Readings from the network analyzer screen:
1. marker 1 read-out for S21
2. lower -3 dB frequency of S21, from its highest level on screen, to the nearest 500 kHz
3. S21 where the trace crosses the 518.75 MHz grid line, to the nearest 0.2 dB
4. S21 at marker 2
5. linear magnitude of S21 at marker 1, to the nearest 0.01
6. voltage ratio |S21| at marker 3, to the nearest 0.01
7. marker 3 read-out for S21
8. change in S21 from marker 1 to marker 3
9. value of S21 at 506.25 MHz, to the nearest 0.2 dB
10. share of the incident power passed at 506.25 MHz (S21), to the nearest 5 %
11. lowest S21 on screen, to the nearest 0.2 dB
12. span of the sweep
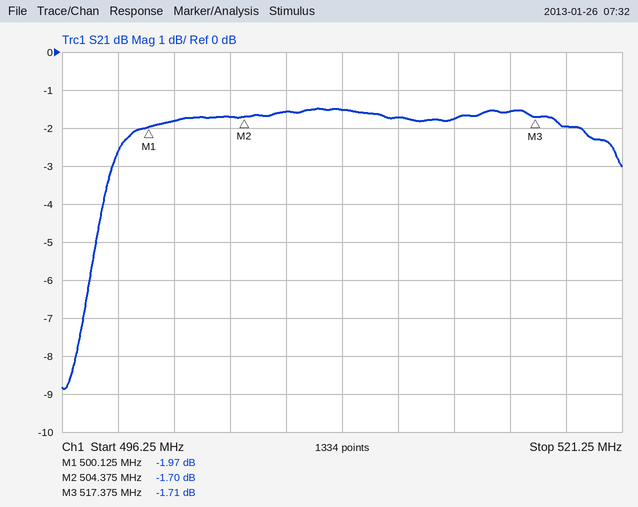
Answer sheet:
-1.97 dB
498.0 MHz
-2.0 dB
-1.70 dB
0.80
0.82
-1.71 dB
0.26 dB
-1.6 dB
70 %
-8.8 dB
25 MHz
